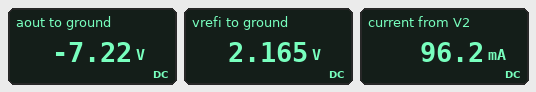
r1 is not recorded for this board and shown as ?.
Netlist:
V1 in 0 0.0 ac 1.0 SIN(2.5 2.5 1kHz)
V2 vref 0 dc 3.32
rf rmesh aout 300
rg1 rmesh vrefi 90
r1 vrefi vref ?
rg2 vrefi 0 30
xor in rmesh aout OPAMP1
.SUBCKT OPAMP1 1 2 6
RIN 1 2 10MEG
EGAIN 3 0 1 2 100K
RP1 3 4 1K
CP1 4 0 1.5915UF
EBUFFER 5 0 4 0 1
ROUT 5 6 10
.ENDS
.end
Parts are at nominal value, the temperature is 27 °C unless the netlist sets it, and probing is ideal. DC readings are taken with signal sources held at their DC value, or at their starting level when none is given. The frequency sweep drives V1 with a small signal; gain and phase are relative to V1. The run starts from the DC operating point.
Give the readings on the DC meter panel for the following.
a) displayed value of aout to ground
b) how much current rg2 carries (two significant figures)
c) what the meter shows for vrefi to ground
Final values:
-7.22 V
72 mA
2.165 V
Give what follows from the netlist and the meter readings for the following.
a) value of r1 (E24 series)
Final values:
12 Ω
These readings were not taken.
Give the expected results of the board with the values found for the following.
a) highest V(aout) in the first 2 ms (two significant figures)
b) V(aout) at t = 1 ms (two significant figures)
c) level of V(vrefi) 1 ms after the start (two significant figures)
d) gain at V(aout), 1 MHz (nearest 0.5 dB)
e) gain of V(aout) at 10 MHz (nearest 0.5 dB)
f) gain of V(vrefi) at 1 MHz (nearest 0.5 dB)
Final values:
13 V
2.9 V
2.4 V
11.5 dB
-0.5 dB
-22.0 dB
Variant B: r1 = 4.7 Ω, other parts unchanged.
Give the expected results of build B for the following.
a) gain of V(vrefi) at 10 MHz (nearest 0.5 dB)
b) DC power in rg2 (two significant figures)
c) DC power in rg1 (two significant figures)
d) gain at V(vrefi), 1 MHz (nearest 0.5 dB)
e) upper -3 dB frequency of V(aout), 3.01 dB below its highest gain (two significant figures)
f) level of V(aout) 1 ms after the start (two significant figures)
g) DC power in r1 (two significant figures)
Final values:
-40.0 dB
250 mW
84 mW
-28.0 dB
2.3 MHz
1.3 V
70 mW
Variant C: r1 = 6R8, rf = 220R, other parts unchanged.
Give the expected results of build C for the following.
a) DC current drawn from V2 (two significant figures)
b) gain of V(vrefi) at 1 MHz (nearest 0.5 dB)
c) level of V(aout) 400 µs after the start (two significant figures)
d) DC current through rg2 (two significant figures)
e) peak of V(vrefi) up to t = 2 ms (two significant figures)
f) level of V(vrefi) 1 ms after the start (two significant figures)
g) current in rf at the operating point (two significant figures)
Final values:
110 mA
-25.0 dB
6.9 V
85 mA
2.8 V
2.7 V
28 mA
